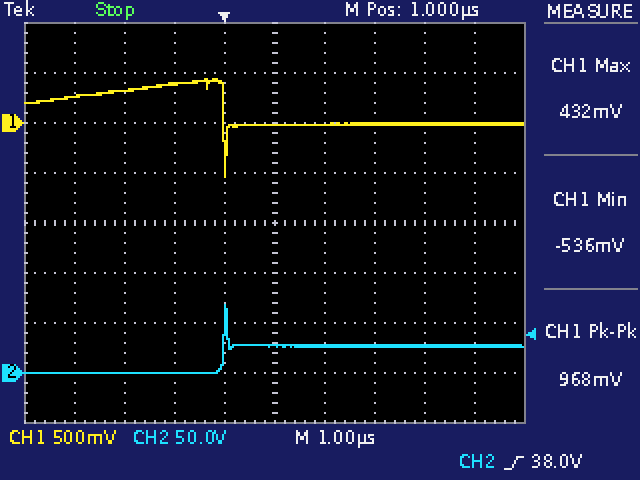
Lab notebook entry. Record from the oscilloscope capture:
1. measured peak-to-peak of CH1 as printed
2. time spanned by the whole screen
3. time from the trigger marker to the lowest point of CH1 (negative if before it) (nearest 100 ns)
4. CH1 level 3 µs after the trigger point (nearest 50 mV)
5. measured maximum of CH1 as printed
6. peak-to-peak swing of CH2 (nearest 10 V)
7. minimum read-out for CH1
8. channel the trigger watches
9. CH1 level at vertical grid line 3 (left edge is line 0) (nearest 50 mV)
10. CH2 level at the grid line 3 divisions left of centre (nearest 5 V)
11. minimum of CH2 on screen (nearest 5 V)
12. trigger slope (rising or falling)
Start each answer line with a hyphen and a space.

- 968 mV
- 10 µs
- 0.0 µs
- 0 mV
- 432 mV
- 70 V
- -536 mV
- CH2
- 400 mV
- 0 V
- 0 V
- rising
